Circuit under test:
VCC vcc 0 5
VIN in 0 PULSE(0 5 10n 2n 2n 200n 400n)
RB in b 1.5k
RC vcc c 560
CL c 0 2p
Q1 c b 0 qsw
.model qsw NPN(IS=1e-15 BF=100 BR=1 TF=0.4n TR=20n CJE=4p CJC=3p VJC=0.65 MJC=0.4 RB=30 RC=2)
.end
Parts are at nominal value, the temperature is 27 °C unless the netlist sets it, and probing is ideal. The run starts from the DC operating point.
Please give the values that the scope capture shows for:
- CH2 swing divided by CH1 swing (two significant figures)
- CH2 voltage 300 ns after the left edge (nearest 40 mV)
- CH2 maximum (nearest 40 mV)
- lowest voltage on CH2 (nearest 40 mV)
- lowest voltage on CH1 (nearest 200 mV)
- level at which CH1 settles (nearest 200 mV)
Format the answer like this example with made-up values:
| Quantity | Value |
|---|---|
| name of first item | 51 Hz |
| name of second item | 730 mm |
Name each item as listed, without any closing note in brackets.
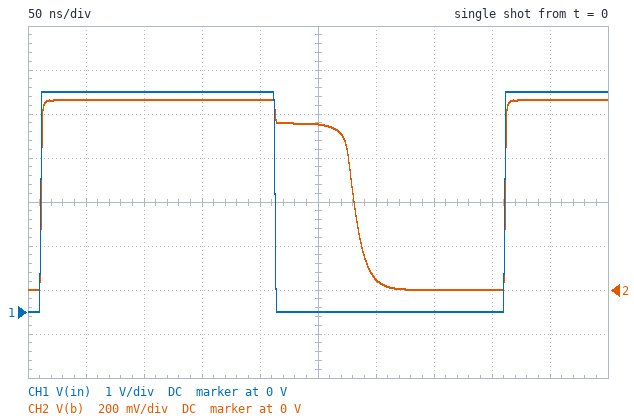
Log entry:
| Quantity | Value |
|---|---|
| CH2 swing divided by CH1 swing | 0.17 |
| CH2 voltage 300 ns after the left edge | 40 mV |
| CH2 maximum | 880 mV |
| lowest voltage on CH2 | 0 V |
| lowest voltage on CH1 | 0 V |
| level at which CH1 settles | 5.0 V |
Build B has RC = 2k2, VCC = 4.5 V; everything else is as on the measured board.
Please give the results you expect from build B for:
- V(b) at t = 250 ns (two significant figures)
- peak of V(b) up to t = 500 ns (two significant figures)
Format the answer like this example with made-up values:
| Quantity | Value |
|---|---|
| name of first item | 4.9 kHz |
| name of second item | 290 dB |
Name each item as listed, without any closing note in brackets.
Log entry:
| Quantity | Value |
|---|---|
| V(b) at t = 250 ns | 710 mV |
| peak of V(b) up to t = 500 ns | 850 mV |
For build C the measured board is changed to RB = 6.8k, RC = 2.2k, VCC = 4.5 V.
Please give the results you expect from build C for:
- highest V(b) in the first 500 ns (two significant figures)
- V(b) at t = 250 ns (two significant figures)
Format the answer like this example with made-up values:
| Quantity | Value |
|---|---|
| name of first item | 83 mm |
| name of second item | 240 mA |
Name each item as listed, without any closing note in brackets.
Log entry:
| Quantity | Value |
|---|---|
| highest V(b) in the first 500 ns | 760 mV |
| V(b) at t = 250 ns | 730 mV |
